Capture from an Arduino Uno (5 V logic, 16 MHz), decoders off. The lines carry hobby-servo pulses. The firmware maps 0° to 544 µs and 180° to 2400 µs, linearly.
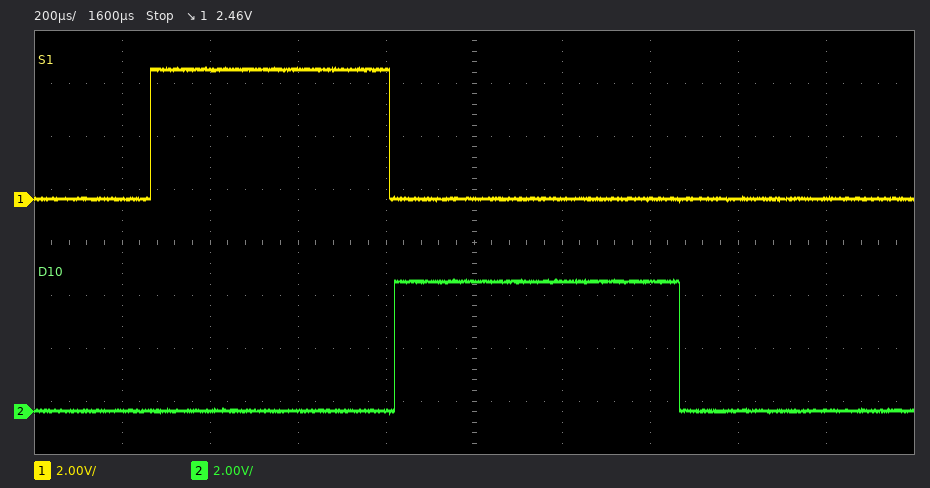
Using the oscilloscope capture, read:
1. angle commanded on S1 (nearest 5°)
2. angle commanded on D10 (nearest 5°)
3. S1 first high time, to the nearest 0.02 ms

0°
10°
0.54 ms
